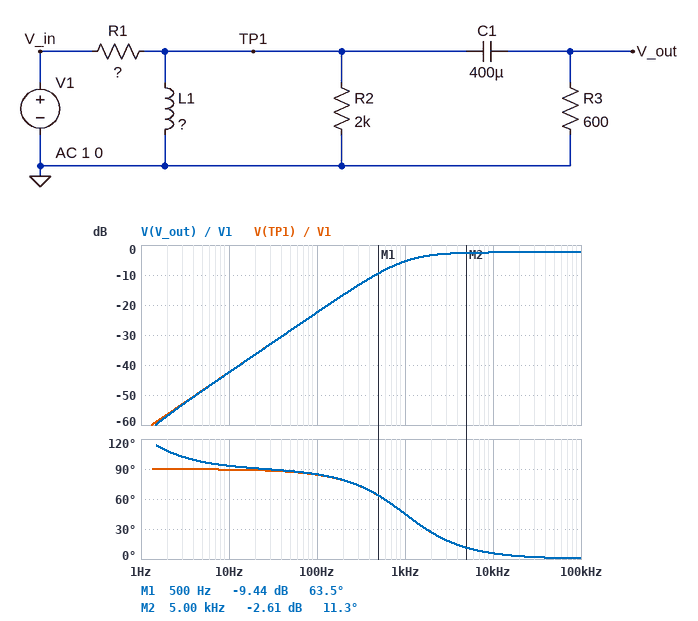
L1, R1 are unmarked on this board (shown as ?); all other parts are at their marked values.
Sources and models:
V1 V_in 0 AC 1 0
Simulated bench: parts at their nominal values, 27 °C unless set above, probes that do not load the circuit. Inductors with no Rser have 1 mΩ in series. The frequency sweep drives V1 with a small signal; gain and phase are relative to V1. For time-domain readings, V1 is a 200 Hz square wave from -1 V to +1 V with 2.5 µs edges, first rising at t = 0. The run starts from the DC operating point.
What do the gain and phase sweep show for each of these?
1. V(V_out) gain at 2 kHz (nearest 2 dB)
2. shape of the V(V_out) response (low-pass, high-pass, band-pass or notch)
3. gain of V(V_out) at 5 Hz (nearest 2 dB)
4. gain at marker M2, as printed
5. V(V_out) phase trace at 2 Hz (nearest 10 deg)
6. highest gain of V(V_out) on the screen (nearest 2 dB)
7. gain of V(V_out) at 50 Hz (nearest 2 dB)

-4 dB
high-pass
-48 dB
-2.61 dB
110 deg
-2 dB
-28 dB
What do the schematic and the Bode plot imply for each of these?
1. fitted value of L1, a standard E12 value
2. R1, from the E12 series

18 mH
150 Ω
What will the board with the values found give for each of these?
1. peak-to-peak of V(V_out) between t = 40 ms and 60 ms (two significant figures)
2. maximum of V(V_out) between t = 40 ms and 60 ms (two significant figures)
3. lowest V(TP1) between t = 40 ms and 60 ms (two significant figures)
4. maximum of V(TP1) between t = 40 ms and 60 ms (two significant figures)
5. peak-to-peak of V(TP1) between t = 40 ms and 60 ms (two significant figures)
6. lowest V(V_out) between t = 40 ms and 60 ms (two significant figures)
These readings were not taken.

3.0 V
1.5 V
-1.5 V
1.5 V
3.0 V
-1.5 V
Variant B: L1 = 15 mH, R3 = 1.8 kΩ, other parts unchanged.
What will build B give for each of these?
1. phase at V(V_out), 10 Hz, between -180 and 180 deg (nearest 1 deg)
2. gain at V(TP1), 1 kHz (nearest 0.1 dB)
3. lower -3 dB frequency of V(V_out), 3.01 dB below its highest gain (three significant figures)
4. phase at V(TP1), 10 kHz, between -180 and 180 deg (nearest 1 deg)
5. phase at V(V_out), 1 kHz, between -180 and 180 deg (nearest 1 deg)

91 deg
-5.9 dB
1.37 kHz
8 deg
54 deg
